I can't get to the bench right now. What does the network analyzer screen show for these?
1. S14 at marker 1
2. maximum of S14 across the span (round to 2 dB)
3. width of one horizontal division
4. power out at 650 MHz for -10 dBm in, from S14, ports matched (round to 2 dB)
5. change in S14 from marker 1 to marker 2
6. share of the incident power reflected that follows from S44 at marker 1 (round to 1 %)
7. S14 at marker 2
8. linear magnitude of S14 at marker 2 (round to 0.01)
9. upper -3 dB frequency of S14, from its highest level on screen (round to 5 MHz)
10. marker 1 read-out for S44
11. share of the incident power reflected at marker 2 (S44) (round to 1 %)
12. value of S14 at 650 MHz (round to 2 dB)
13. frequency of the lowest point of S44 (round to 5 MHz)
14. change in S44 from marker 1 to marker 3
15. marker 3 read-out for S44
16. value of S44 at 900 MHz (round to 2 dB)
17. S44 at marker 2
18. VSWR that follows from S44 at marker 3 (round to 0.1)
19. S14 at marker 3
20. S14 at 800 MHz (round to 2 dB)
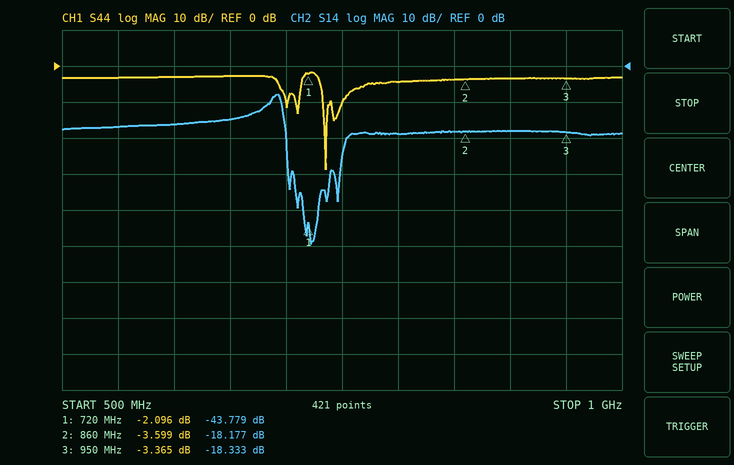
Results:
-43.779 dB
-8 dB
50 MHz
-24 dBm
25.602 dB
62 %
-18.177 dB
0.12
695 MHz
-2.096 dB
44 %
-14 dB
735 MHz
-1.269 dB
-3.365 dB
-4 dB
-3.599 dB
5.2
-18.333 dB
-18 dB
